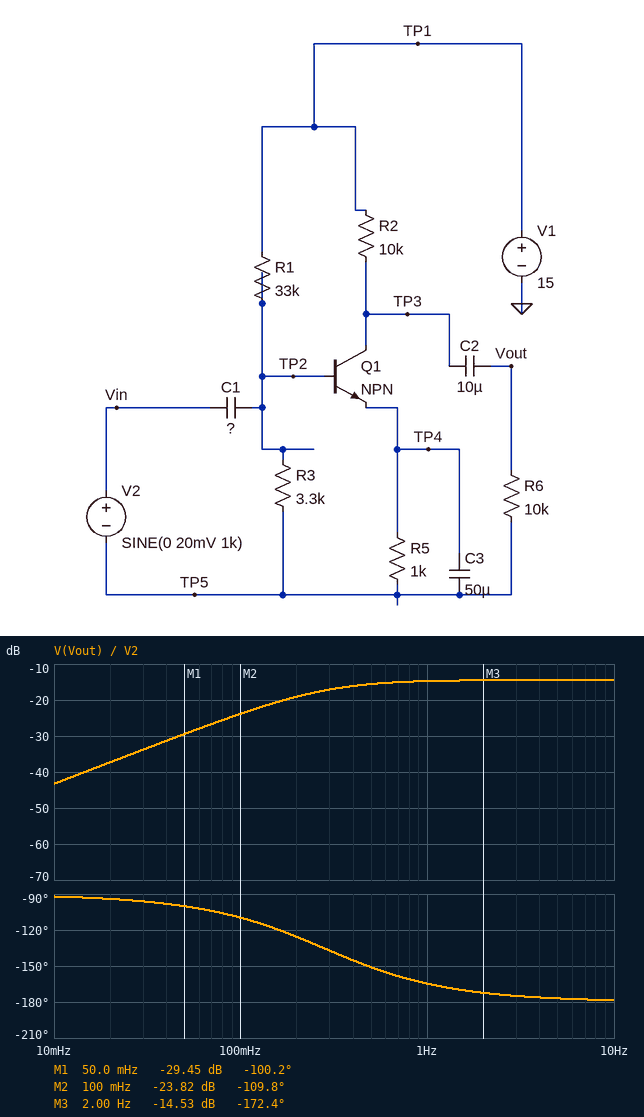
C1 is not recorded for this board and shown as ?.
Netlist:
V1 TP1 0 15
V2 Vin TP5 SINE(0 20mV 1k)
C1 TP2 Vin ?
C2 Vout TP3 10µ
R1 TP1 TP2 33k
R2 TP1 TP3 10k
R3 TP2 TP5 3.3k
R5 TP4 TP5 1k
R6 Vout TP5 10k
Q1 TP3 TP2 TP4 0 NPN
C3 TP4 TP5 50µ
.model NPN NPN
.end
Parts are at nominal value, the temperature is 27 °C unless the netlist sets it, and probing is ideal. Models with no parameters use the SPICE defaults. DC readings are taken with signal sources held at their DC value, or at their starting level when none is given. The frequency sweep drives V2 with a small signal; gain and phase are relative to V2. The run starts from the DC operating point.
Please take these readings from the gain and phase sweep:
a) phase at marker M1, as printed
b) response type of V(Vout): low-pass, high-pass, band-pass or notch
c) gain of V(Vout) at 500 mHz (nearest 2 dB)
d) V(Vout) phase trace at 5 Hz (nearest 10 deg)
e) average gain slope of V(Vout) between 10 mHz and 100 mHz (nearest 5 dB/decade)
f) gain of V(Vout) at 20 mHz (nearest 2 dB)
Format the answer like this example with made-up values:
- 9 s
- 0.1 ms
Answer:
- -100.2 deg
- high-pass
- -16 dB
- -180 deg
- 20 dB/decade
- -38 dB
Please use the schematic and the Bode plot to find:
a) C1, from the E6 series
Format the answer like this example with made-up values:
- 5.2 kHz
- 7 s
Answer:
- 33 µF
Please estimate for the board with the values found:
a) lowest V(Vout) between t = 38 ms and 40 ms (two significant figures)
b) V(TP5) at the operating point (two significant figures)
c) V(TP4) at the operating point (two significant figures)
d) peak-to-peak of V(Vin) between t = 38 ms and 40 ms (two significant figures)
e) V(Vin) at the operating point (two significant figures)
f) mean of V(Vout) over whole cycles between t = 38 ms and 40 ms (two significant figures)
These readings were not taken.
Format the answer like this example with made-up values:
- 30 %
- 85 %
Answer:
- 15 V
- 15 V
- 15 V
- 25 mV
- 15 V
- 15 V
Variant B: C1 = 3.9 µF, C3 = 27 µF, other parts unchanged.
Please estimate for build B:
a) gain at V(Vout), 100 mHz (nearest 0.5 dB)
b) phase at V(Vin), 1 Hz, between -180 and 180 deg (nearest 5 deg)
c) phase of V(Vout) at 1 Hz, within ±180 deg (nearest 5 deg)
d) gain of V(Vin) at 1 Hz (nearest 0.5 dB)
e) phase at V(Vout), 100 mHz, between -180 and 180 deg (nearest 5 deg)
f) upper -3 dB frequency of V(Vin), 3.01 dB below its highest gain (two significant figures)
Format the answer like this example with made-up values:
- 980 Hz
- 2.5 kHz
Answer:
- -42.5 dB
- 0 deg
- -135 deg
- 0 dB
- -105 deg
- 27 Hz
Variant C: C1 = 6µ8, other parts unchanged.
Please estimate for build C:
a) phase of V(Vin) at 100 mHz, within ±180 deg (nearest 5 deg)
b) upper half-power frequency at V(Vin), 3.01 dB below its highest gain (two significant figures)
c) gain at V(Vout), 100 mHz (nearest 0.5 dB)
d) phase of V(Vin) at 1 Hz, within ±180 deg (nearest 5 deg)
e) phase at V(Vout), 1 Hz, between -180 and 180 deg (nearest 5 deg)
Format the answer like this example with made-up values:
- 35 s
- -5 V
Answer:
- 0 deg
- 15 Hz
- -37.5 dB
- -5 deg
- -140 deg
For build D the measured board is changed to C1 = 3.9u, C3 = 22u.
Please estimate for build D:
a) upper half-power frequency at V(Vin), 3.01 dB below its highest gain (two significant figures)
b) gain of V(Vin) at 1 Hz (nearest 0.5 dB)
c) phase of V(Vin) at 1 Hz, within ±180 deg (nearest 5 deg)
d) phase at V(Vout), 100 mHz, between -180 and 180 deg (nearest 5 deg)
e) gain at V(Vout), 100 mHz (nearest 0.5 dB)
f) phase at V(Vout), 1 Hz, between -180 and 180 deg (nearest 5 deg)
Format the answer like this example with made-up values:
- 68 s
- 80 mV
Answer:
- 27 Hz
- 0 dB
- 0 deg
- -105 deg
- -42.5 dB
- -135 deg
